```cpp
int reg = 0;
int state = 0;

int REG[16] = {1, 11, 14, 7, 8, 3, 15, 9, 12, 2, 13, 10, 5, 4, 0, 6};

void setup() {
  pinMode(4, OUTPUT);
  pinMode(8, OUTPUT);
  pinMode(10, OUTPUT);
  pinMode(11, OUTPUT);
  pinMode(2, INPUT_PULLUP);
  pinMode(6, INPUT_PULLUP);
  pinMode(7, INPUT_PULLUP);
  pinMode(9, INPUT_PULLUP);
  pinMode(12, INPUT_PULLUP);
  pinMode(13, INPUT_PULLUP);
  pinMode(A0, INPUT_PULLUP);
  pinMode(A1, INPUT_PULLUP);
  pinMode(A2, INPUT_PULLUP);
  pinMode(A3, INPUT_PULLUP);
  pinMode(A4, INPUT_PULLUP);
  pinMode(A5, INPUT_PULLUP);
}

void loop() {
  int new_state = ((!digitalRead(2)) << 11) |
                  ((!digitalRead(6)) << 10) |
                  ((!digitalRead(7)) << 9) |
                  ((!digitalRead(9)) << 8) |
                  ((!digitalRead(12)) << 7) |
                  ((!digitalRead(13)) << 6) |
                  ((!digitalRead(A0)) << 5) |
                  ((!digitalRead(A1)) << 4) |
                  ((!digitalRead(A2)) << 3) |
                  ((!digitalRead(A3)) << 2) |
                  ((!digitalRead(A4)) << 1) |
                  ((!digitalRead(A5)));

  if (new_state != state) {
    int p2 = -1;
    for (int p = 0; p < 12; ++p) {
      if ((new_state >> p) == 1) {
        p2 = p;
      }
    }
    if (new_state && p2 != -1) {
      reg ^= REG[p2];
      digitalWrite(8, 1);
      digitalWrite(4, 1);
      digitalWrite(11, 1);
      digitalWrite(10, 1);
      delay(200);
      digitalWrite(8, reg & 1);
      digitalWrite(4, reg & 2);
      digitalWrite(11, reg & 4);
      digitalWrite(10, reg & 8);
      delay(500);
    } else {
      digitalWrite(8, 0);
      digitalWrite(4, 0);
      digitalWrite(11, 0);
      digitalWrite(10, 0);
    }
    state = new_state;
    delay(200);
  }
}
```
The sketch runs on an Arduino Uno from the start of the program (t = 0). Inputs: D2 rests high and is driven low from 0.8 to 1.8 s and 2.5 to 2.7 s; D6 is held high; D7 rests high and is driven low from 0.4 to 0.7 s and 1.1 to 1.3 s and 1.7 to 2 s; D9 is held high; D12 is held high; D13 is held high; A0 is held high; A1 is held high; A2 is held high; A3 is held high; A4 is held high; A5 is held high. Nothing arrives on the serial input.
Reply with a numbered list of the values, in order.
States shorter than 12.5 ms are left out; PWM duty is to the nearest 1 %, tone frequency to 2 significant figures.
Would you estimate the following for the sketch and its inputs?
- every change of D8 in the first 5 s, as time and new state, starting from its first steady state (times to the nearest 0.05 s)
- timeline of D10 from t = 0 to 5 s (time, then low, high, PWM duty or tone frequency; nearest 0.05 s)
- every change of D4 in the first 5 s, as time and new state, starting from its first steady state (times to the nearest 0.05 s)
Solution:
1. 0 s low; 0.4 s high; 0.6 s low; 1.3 s high; 1.5 s low; 2.5 s high; 2.7 s low
2. 0 s low; 0.4 s high; 0.6 s low; 1.3 s high; 2.2 s low; 2.5 s high; 2.7 s low
3. 0 s low; 0.4 s high; 1.5 s low; 2.5 s high; 3.4 s low
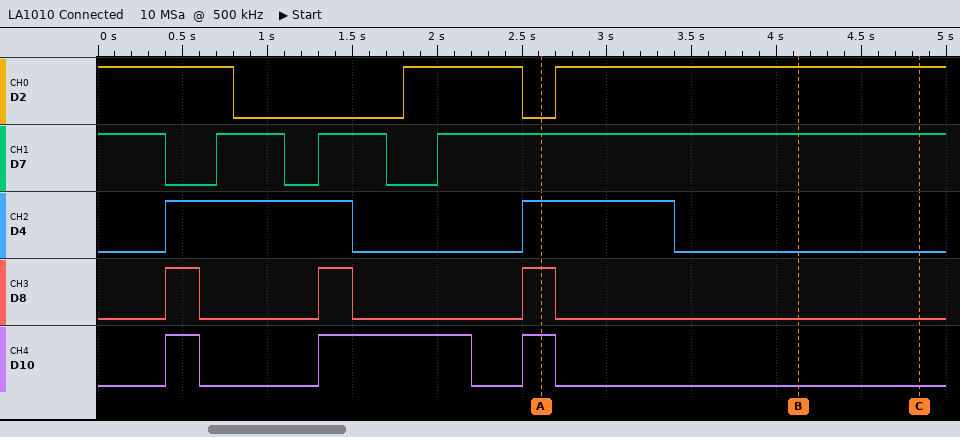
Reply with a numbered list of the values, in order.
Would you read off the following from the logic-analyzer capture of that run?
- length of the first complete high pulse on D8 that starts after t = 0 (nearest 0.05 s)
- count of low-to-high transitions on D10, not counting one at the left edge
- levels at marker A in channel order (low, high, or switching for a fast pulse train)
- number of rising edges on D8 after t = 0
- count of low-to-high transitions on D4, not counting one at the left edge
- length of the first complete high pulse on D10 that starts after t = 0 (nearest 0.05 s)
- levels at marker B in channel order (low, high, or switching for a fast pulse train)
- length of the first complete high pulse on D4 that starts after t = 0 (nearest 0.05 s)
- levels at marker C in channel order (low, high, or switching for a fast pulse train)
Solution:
1. 0.20 s
2. 3
3. D2 low, D7 high, D4 high, D8 high, D10 high
4. 3
5. 2
6. 0.20 s
7. D2 high, D7 high, D4 low, D8 low, D10 low
8. 1.10 s
9. D2 high, D7 high, D4 low, D8 low, D10 low
